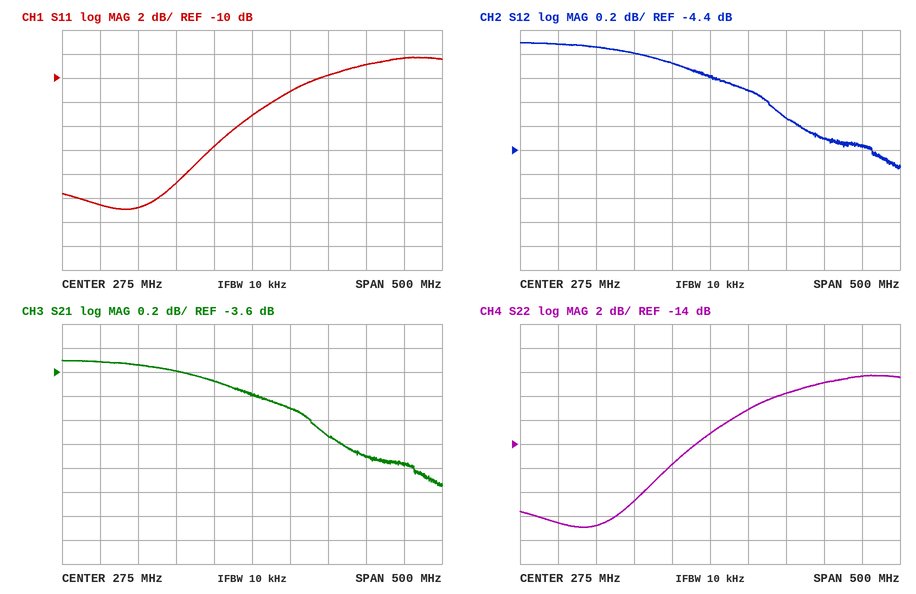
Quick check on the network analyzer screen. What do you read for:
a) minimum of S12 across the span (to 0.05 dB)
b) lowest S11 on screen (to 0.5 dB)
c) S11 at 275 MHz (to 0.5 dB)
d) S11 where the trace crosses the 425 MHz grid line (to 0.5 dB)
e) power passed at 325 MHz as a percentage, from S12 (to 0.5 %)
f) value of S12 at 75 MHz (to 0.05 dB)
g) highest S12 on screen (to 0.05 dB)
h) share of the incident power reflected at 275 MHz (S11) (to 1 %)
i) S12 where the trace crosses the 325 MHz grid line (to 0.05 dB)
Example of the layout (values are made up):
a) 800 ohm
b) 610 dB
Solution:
a) -4.55 dB
b) -21.0 dB
c) -13.0 dB
d) -9.0 dB
e) 40.5 %
f) -3.50 dB
g) -3.50 dB
h) 5 %
i) -3.90 dB
